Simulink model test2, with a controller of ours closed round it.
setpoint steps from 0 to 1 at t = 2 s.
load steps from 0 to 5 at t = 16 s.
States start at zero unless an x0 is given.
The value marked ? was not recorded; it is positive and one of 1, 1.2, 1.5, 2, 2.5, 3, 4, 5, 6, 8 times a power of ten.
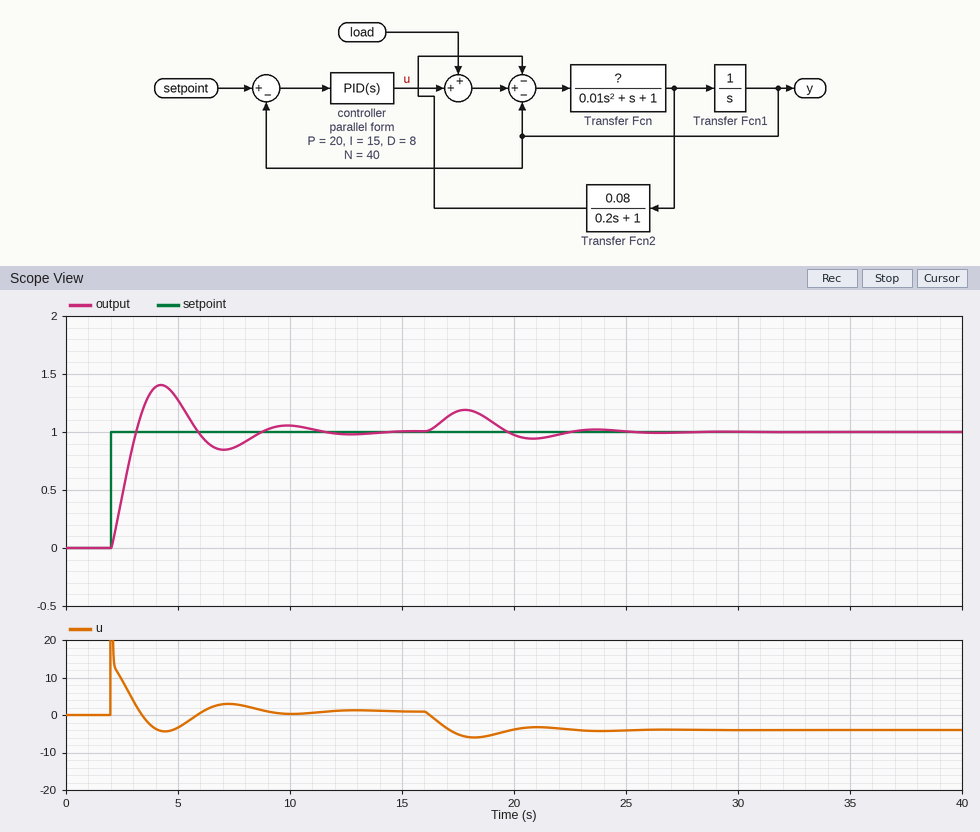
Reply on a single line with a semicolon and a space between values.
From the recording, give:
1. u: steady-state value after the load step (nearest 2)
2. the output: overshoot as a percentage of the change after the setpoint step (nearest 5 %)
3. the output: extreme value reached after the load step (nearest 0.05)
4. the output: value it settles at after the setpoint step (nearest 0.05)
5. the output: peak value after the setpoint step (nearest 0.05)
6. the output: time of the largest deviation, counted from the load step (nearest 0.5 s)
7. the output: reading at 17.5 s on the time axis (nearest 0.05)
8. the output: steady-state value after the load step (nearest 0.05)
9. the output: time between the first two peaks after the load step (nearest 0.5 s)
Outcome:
-4; 40 %; 1.20; 1.00; 1.40; 2.0 s; 1.20; 1.00; 6.0 s
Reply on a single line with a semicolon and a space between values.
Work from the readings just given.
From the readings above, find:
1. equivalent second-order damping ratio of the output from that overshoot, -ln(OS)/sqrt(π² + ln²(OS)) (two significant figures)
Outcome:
0.28
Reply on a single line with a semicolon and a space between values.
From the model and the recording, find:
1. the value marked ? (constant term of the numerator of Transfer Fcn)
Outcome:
0.1
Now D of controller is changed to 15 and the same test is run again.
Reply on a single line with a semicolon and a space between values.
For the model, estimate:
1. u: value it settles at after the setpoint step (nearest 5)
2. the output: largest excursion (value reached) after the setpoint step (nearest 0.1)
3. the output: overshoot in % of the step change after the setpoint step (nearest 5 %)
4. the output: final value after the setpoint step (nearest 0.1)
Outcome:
0; 1.2; 25 %; 1.0
